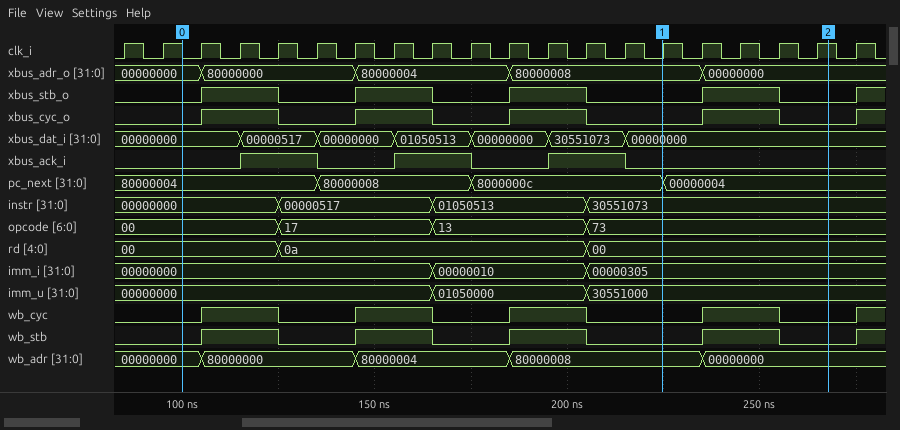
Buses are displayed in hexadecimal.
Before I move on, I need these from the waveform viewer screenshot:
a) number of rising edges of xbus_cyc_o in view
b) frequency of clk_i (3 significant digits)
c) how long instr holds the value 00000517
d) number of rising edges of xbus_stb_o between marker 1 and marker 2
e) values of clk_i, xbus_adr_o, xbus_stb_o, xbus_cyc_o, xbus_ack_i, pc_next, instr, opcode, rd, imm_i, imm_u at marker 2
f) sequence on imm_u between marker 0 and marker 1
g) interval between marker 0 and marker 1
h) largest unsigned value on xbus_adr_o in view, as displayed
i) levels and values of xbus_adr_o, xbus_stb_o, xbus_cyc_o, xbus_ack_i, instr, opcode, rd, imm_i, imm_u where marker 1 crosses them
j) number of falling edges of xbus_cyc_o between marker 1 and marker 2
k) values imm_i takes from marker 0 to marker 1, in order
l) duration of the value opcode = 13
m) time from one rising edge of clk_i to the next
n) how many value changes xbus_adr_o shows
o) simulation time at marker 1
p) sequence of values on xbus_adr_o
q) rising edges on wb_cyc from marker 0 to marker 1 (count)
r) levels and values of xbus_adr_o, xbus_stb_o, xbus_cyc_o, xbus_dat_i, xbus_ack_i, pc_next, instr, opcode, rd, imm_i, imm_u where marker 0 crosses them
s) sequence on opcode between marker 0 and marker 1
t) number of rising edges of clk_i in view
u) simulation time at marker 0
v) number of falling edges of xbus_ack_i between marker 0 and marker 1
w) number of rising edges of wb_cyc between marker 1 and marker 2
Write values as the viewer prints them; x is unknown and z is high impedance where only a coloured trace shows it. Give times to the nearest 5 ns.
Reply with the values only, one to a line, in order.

5
100 MHz
40 ns
1
clk_i=1, xbus_adr_o=00000000, xbus_stb_o=0, xbus_cyc_o=0, xbus_ack_i=0, pc_next=00000004, instr=30551073, opcode=73, rd=00, imm_i=00000305, imm_u=30551000
00000000, 01050000, 30551000
125 ns
80000008
xbus_adr_o=80000008, xbus_stb_o=0, xbus_cyc_o=0, xbus_ack_i=0, instr=30551073, opcode=73, rd=00, imm_i=00000305, imm_u=30551000
1
00000000, 00000010, 00000305
40 ns
10 ns
4
225 ns
00000000, 80000000, 80000004, 80000008, 00000000
3
xbus_adr_o=00000000, xbus_stb_o=0, xbus_cyc_o=0, xbus_dat_i=00000000, xbus_ack_i=0, pc_next=80000004, instr=00000000, opcode=00, rd=00, imm_i=00000000, imm_u=00000000
00, 17, 13, 73
20
100 ns
3
1
